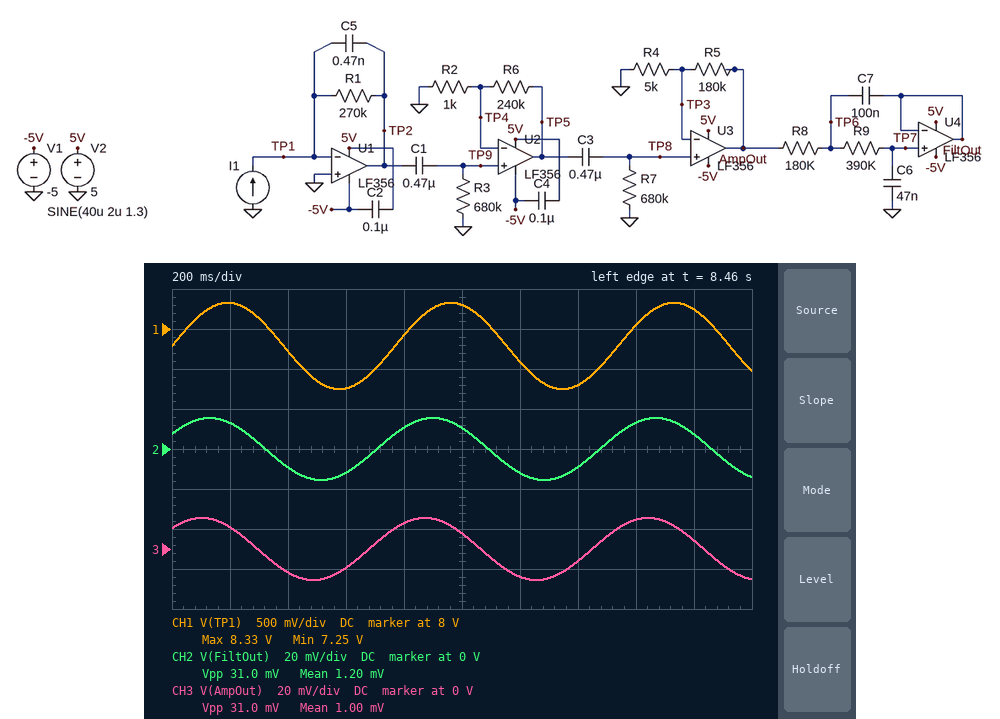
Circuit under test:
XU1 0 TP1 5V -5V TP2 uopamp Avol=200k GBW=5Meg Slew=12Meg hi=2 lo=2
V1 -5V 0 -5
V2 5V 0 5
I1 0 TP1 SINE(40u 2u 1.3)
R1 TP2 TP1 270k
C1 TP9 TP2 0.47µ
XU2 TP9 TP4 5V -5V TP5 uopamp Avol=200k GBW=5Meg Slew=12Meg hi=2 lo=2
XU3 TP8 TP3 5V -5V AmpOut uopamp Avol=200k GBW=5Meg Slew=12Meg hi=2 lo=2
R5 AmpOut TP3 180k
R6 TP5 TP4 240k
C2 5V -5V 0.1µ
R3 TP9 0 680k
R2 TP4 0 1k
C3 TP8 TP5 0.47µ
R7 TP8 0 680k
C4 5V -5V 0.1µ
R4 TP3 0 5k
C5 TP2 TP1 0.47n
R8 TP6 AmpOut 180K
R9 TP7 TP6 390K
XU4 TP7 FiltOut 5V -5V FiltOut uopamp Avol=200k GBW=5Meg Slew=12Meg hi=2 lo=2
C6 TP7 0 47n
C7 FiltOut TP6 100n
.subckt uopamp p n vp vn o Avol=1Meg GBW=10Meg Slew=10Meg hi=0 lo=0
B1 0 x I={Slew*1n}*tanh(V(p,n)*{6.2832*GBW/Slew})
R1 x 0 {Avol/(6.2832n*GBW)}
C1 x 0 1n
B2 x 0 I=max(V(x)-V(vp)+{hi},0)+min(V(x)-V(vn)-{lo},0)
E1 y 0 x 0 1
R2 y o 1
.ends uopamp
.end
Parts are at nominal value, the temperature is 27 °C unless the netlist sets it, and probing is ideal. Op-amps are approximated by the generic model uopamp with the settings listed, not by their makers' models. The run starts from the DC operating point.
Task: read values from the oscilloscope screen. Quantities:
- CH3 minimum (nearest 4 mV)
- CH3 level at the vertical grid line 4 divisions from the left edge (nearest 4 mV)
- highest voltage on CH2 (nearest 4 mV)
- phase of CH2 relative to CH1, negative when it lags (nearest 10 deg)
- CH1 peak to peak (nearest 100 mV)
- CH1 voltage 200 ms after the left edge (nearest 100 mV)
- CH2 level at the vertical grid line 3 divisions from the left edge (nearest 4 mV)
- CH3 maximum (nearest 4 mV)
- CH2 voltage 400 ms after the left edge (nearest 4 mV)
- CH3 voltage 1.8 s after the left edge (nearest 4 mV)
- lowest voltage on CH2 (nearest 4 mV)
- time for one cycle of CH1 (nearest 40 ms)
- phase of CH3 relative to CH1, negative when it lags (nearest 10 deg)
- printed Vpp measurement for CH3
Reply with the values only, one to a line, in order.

-16 mV
12 mV
16 mV
30 deg
1.1 V
8.3 V
-12 mV
16 mV
-8 mV
4 mV
-16 mV
760 ms
40 deg
31.0 mV
